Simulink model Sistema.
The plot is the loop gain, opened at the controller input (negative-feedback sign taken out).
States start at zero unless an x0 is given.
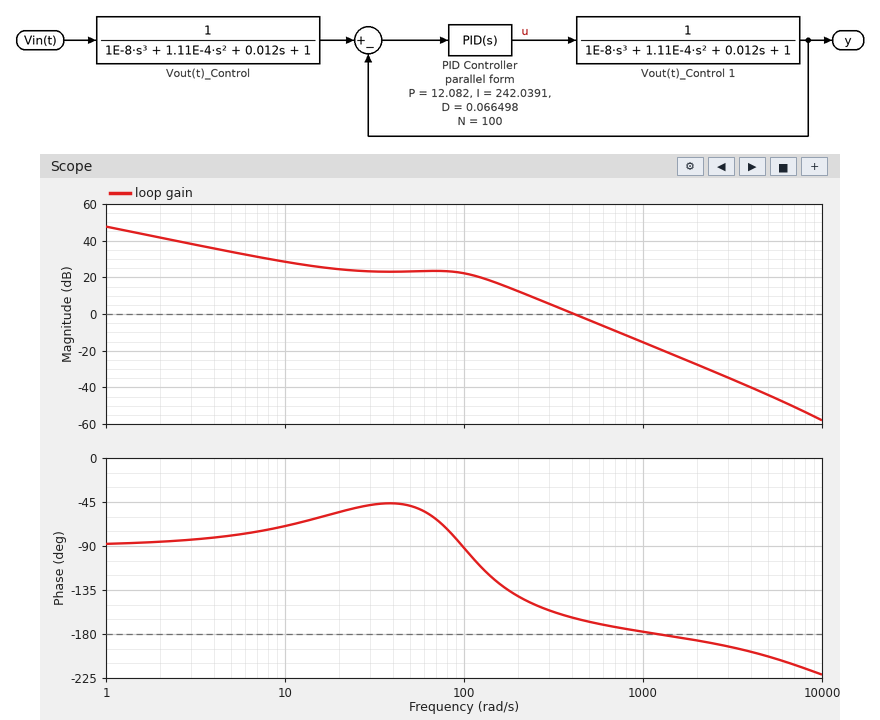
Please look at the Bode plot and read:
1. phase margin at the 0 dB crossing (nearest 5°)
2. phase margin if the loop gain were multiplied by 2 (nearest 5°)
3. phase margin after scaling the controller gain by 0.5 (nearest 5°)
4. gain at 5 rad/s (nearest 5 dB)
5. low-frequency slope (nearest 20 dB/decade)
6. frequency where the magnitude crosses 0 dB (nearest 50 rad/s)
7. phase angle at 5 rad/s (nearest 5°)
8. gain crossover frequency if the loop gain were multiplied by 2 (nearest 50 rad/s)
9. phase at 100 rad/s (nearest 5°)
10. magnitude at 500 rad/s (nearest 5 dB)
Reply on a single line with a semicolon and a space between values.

15°; 10°; 25°; 35 dB; -20 dB/decade; 400 rad/s; -80°; 600 rad/s; -90°; -5 dB
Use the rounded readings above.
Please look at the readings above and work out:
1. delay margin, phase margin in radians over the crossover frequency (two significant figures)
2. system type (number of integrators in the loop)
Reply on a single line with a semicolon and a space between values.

0.00065 s; 1
